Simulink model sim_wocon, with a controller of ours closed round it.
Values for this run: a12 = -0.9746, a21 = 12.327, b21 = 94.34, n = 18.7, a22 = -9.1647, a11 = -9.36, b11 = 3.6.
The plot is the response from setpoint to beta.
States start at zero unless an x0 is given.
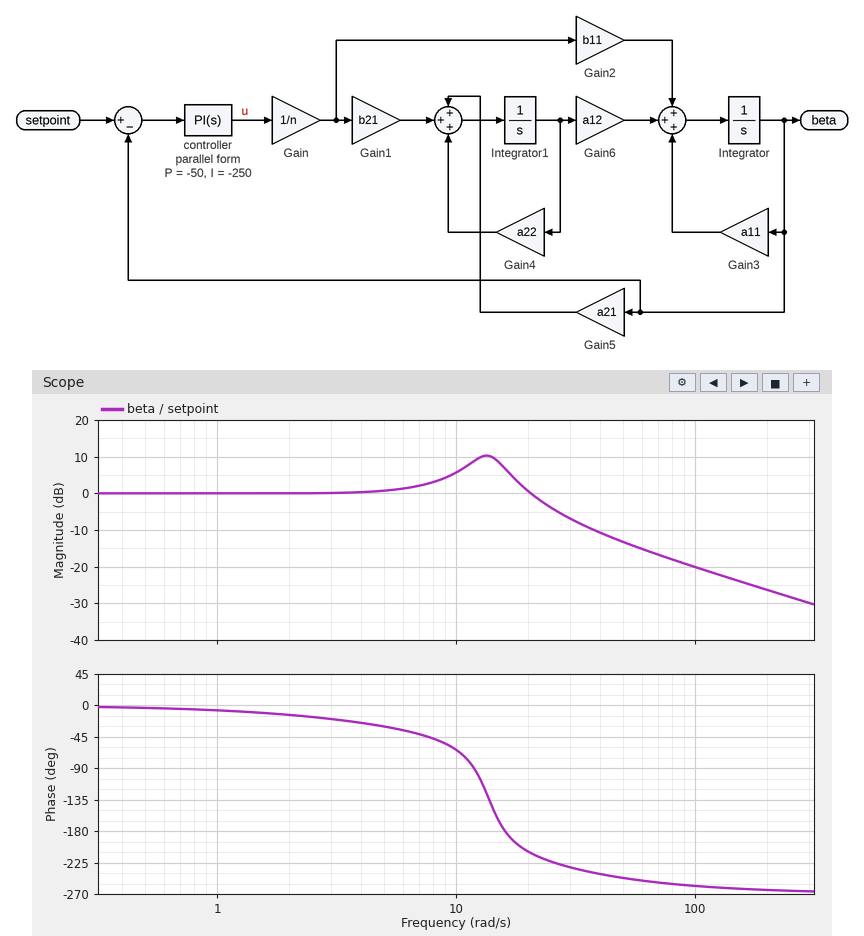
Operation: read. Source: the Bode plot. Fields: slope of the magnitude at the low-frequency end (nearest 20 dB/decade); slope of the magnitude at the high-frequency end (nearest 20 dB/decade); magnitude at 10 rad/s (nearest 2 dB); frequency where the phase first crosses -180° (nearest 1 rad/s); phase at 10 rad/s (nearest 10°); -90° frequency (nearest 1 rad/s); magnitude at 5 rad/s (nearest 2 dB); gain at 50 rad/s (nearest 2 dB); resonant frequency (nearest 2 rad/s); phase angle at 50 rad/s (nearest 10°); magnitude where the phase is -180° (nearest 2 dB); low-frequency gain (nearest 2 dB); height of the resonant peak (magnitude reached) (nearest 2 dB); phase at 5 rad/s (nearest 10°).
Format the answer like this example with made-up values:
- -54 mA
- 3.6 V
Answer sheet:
- 0 dB/decade
- -20 dB/decade
- 6 dB
- 16 rad/s
- -60°
- 12 rad/s
- 0 dB
- -14 dB
- 14 rad/s
- -250°
- 6 dB
- 0 dB
- 10 dB
- -30°
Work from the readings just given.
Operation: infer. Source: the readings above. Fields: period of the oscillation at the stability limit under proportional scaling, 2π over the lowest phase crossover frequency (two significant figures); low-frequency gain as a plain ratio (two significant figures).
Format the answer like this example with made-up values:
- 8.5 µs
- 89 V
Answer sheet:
- 0.39 s
- 1.0
